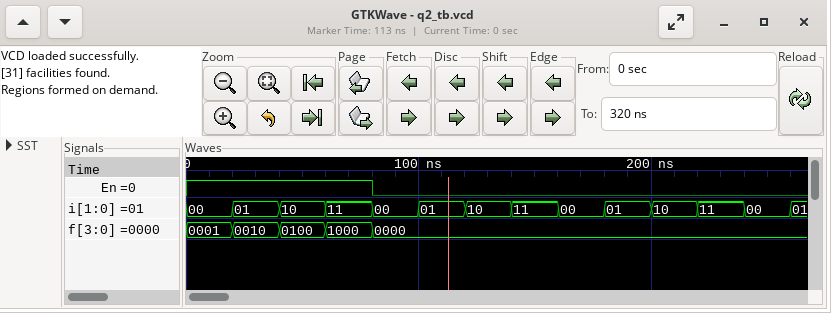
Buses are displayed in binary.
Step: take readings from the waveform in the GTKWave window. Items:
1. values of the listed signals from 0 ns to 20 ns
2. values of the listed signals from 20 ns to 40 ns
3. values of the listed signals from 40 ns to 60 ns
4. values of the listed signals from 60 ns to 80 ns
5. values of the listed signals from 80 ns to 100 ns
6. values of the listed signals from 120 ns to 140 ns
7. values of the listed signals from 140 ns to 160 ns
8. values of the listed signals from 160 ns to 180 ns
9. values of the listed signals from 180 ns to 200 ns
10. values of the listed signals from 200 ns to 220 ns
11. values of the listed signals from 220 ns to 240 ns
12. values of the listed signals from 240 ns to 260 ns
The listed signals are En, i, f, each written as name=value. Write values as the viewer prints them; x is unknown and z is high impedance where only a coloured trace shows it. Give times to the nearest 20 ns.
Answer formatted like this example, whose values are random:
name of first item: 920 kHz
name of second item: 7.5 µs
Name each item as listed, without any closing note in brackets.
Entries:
values of the listed signals from 0 ns to 20 ns: En=1, i=00, f=0001
values of the listed signals from 20 ns to 40 ns: En=1, i=01, f=0010
values of the listed signals from 40 ns to 60 ns: En=1, i=10, f=0100
values of the listed signals from 60 ns to 80 ns: En=1, i=11, f=1000
values of the listed signals from 80 ns to 100 ns: En=0, i=00, f=0000
values of the listed signals from 120 ns to 140 ns: En=0, i=10, f=0000
values of the listed signals from 140 ns to 160 ns: En=0, i=11, f=0000
values of the listed signals from 160 ns to 180 ns: En=0, i=00, f=0000
values of the listed signals from 180 ns to 200 ns: En=0, i=01, f=0000
values of the listed signals from 200 ns to 220 ns: En=0, i=10, f=0000
values of the listed signals from 220 ns to 240 ns: En=0, i=11, f=0000
values of the listed signals from 240 ns to 260 ns: En=0, i=00, f=0000
